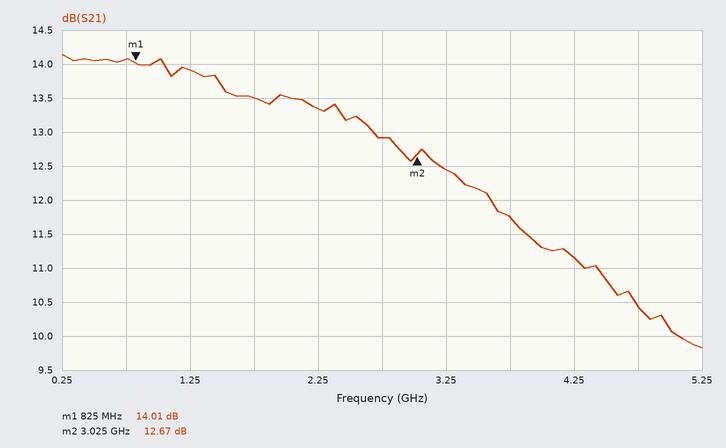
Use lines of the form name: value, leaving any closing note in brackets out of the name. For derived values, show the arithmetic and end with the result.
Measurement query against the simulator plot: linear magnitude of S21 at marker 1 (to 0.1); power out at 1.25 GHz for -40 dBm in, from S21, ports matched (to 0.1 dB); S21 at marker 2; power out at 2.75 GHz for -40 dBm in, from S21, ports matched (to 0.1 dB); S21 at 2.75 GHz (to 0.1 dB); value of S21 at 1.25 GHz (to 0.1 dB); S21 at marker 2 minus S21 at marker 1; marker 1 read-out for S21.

linear magnitude of S21 at marker 1: 10^(14.01/20) ≈ 5.0
power out at 1.25 GHz for -40 dBm in, from S21, ports matched: -40 dBm + (13.9 dB) = -26.1 dBm
S21 at marker 2: 12.67 dB
power out at 2.75 GHz for -40 dBm in, from S21, ports matched: -40 dBm + (12.9 dB) = -27.1 dBm
S21 at 2.75 GHz: 12.9 dB
value of S21 at 1.25 GHz: 13.9 dB
S21 at marker 2 minus S21 at marker 1: 12.67 − (14.01) = -1.34 dB
marker 1 read-out for S21: 14.01 dB
